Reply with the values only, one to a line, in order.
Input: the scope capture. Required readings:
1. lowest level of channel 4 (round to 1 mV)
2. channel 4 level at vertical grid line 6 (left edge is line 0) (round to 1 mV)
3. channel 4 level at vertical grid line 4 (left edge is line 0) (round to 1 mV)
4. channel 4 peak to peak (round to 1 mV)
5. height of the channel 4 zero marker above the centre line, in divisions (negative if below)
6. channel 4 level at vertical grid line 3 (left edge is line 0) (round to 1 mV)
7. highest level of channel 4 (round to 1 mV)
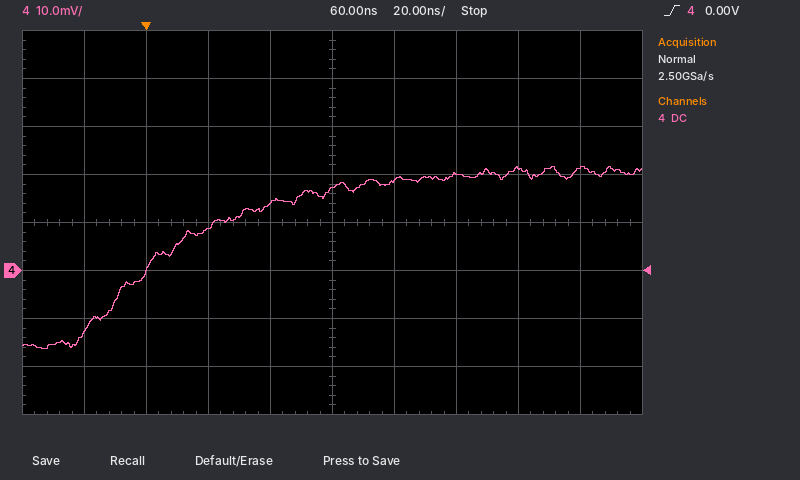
-16 mV
19 mV
14 mV
38 mV
-1.0 div
9 mV
22 mV
